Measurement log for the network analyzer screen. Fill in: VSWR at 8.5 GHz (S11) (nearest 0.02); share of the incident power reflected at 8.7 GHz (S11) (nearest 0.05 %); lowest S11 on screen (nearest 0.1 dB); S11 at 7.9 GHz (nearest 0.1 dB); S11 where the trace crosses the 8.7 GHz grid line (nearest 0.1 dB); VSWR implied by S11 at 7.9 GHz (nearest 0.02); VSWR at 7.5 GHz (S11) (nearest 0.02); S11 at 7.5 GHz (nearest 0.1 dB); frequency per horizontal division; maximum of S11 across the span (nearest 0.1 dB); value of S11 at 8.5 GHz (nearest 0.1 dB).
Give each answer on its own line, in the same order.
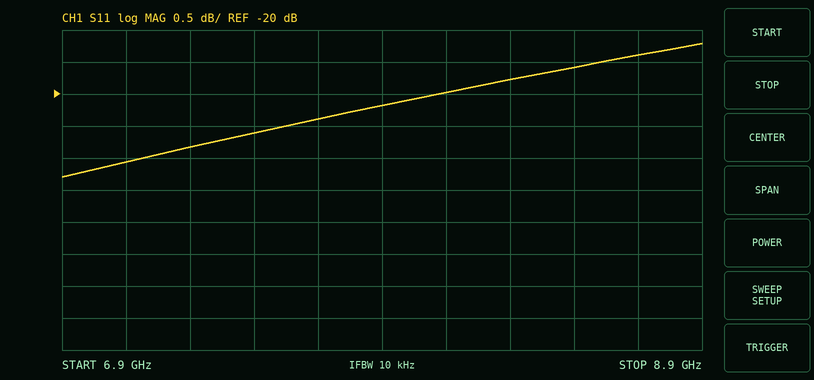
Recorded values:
1.24
1.15 %
-21.3 dB
-20.2 dB
-19.4 dB
1.22
1.20
-20.6 dB
200 MHz
-19.2 dB
-19.6 dB
